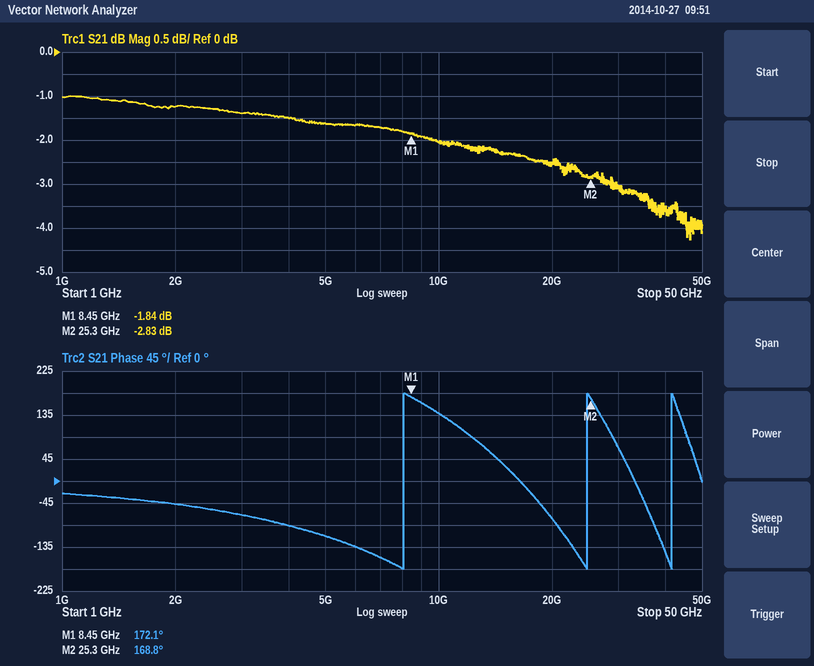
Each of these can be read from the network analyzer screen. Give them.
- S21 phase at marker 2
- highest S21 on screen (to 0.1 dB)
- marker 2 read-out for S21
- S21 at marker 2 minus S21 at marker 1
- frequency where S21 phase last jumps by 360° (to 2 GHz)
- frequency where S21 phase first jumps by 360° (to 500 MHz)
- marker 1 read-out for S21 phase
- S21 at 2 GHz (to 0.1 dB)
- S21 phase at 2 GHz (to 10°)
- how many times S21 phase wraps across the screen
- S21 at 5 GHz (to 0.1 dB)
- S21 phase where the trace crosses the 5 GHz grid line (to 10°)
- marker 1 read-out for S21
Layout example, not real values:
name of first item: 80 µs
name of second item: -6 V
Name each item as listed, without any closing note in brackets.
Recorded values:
S21 phase at marker 2: 168.8°
highest S21 on screen: -1.0 dB
marker 2 read-out for S21: -2.83 dB
S21 at marker 2 minus S21 at marker 1: -0.99 dB
frequency where S21 phase last jumps by 360°: 42 GHz
frequency where S21 phase first jumps by 360°: 8.0 GHz
marker 1 read-out for S21 phase: 172.1°
S21 at 2 GHz: -1.2 dB
S21 phase at 2 GHz: -50°
how many times S21 phase wraps across the screen: 3
S21 at 5 GHz: -1.6 dB
S21 phase where the trace crosses the 5 GHz grid line: -110°
marker 1 read-out for S21: -1.84 dB
